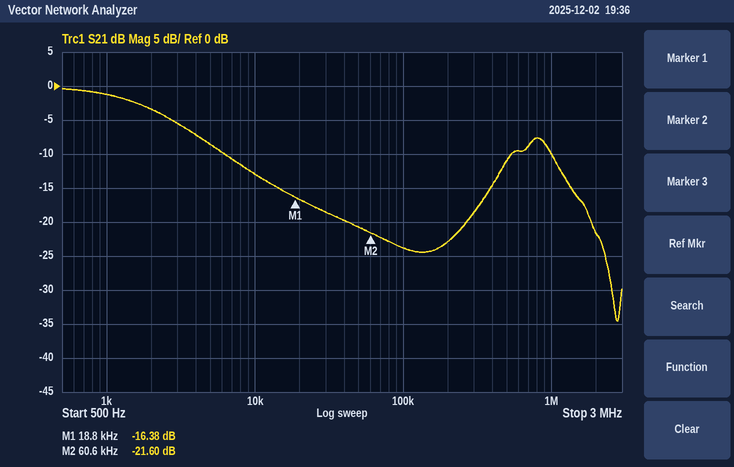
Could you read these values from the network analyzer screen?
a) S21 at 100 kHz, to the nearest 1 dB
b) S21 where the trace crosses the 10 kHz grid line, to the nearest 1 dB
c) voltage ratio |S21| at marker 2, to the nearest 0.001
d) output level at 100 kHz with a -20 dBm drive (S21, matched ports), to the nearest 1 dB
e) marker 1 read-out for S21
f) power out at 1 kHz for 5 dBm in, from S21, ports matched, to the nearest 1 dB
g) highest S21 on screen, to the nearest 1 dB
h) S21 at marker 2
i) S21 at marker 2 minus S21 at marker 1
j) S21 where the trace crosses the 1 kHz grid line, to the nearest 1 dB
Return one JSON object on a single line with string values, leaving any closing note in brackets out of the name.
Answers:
{"S21 at 100 kHz, to the nearest 1 dB": "-24 dB", "S21 where the trace crosses the 10 kHz grid line, to the nearest 1 dB": "-13 dB", "voltage ratio |S21| at marker 2, to the nearest 0.001": "0.083", "output level at 100 kHz with a -20 dBm drive (S21, matched ports), to the nearest 1 dB": "-44 dBm", "marker 1 read-out for S21": "-16.38 dB", "power out at 1 kHz for 5 dBm in, from S21, ports matched, to the nearest 1 dB": "4 dBm", "highest S21 on screen, to the nearest 1 dB": "0 dB", "S21 at marker 2": "-21.60 dB", "S21 at marker 2 minus S21 at marker 1": "-5.22 dB", "S21 where the trace crosses the 1 kHz grid line, to the nearest 1 dB": "-1 dB"}
